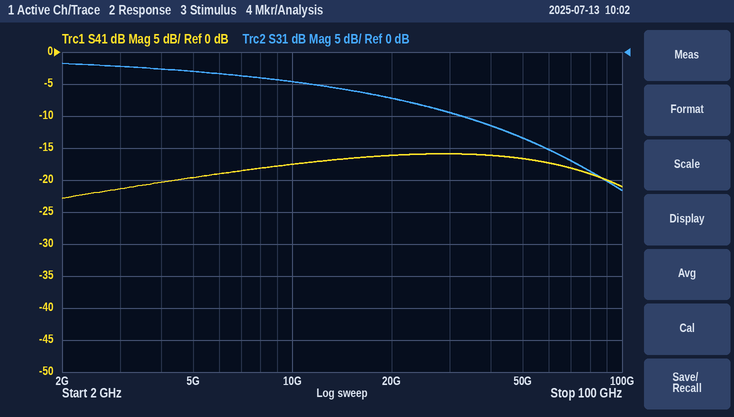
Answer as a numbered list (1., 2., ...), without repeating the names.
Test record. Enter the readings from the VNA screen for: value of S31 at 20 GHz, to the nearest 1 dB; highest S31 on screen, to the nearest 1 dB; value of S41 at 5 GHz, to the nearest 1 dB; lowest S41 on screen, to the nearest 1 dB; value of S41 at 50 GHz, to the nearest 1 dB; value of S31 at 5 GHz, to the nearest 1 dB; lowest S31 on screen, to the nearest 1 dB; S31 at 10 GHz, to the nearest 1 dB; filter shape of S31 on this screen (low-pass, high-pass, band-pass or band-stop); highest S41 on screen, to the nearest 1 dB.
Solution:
1. -7 dB
2. -2 dB
3. -20 dB
4. -23 dB
5. -17 dB
6. -3 dB
7. -22 dB
8. -5 dB
9. low-pass
10. -16 dB
